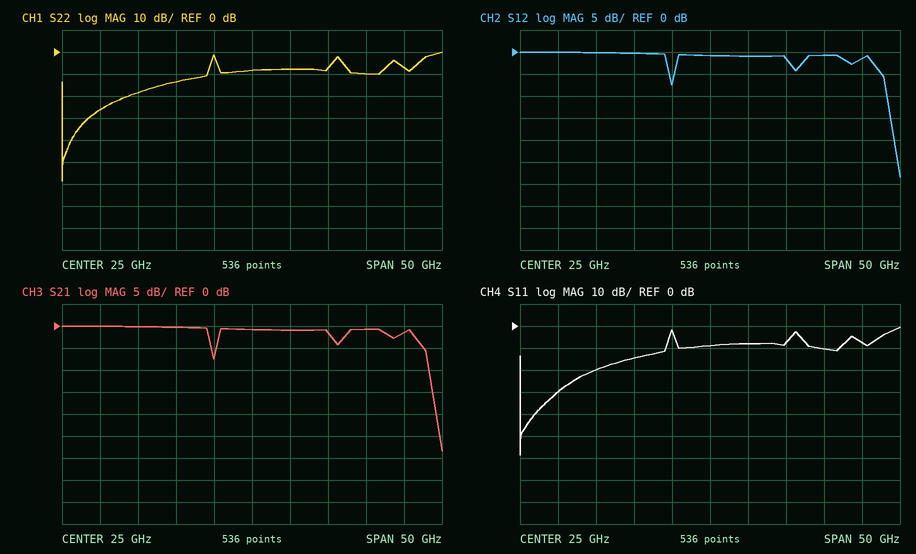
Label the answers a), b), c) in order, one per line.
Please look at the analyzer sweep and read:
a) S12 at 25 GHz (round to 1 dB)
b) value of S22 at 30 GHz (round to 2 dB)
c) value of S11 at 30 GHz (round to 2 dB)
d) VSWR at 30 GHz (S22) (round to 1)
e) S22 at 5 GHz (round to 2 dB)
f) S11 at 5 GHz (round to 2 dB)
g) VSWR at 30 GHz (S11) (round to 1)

a) -1 dB
b) -8 dB
c) -8 dB
d) 2
e) -26 dB
f) -30 dB
g) 2
